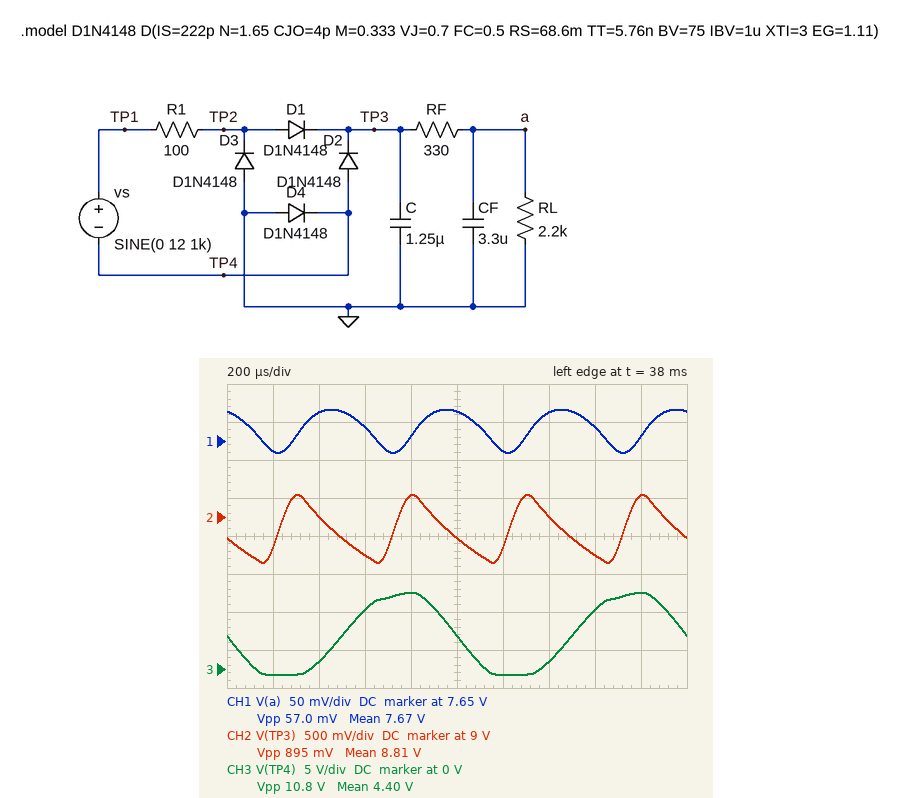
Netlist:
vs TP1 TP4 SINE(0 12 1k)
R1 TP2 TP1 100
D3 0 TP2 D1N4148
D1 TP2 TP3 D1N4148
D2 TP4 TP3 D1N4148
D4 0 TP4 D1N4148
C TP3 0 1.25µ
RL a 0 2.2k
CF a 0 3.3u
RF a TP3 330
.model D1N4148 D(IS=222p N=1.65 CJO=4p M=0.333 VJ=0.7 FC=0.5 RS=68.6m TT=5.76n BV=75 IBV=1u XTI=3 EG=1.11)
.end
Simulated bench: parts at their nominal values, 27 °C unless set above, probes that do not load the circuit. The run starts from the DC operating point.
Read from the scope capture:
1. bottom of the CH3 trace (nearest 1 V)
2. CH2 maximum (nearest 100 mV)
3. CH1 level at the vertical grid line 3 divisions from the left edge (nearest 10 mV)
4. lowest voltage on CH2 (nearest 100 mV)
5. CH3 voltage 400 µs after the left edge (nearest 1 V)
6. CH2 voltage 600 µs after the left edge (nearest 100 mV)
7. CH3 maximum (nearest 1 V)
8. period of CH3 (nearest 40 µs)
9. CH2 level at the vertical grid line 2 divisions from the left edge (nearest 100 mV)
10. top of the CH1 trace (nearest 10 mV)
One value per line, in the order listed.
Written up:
-1 V
9.3 V
7.67 V
8.4 V
1 V
8.5 V
10 V
1.00 ms
9.0 V
7.69 V
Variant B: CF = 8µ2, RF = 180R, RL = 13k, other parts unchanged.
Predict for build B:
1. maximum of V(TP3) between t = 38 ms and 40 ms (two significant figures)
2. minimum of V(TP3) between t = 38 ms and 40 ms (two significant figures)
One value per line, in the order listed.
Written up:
10 V
9.9 V
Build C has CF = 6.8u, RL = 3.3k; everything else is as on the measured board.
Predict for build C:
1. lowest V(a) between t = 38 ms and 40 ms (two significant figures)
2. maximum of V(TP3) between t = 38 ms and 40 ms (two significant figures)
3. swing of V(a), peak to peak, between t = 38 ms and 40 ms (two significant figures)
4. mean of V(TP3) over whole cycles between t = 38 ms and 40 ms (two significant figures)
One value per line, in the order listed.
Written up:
8.3 V
9.5 V
21 mV
9.2 V
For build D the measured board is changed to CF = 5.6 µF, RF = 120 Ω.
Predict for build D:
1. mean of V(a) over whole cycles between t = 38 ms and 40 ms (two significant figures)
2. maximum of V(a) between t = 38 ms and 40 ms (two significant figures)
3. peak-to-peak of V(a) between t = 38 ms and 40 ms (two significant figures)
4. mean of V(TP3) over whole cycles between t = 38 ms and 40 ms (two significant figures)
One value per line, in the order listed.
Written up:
8.2 V
8.3 V
86 mV
8.7 V
